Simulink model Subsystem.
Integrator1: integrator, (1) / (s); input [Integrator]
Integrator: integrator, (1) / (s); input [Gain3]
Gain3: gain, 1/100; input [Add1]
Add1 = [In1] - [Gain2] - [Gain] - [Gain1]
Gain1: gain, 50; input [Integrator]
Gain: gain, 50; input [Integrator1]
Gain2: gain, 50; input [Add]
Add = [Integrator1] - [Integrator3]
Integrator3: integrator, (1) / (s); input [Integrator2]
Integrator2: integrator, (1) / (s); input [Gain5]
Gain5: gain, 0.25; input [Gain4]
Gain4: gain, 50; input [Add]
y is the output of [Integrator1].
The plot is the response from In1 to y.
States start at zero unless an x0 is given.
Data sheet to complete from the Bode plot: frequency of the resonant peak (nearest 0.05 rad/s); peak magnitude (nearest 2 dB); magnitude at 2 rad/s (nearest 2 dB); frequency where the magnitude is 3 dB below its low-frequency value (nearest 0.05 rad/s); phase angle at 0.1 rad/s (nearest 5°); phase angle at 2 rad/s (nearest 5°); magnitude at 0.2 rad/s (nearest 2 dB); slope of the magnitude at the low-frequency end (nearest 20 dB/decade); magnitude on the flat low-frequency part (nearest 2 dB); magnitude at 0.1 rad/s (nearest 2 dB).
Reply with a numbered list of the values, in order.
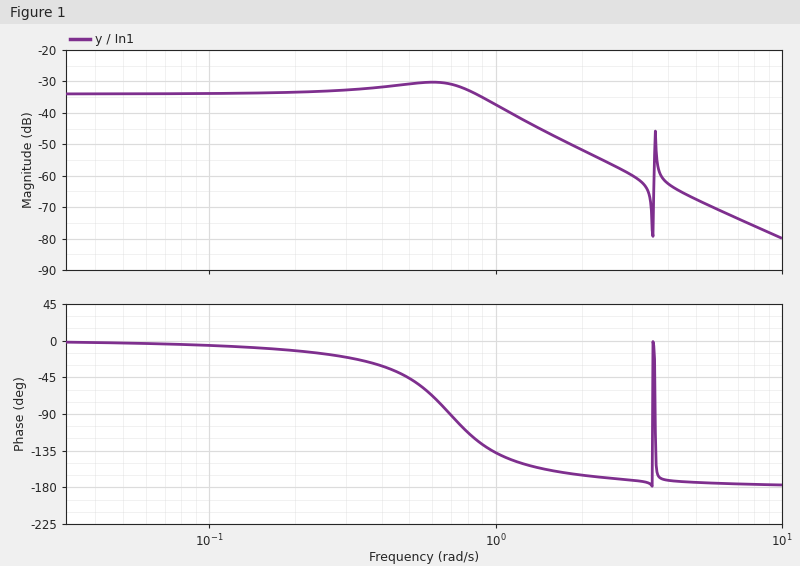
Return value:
1. 0.60 rad/s
2. -30 dB
3. -52 dB
4. 1.00 rad/s
5. -5°
6. -165°
7. -34 dB
8. 0 dB/decade
9. -34 dB
10. -34 dB
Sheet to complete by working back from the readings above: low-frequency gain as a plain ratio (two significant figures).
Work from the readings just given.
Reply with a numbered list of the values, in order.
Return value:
1. 0.020
